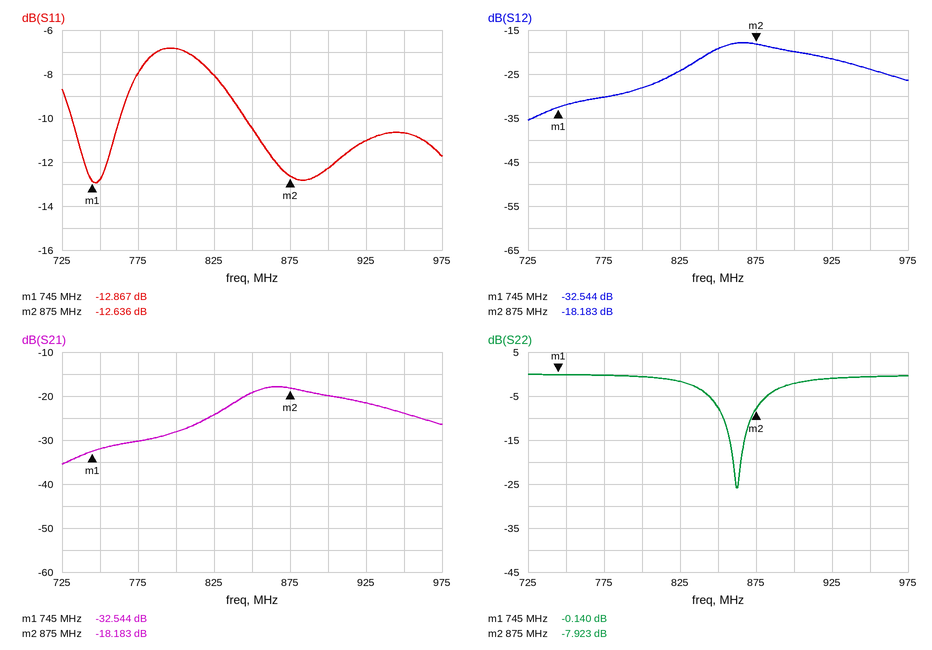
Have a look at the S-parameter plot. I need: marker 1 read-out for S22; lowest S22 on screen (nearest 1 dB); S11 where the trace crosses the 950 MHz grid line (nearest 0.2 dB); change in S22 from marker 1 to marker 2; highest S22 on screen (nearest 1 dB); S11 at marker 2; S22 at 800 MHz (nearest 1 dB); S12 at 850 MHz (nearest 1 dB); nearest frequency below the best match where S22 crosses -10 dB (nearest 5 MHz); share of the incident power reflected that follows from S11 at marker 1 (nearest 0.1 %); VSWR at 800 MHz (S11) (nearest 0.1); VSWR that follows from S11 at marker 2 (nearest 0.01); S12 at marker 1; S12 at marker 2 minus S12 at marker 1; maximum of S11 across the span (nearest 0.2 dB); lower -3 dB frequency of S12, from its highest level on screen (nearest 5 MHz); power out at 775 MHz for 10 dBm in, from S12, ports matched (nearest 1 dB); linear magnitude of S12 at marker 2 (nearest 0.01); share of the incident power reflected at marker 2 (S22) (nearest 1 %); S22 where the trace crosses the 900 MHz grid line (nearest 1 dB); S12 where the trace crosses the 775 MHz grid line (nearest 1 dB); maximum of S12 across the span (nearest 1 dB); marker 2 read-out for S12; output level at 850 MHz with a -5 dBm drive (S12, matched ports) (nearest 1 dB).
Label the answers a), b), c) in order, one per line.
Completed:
a) -0.140 dB
b) -26 dB
c) -10.6 dB
d) -7.783 dB
e) 0 dB
f) -12.636 dB
g) -1 dB
h) -19 dB
i) 855 MHz
j) 5.2 %
k) 2.7
l) 1.61
m) -32.544 dB
n) 14.361 dB
o) -6.8 dB
p) 840 MHz
q) -20 dBm
r) 0.12
s) 16 %
t) -2 dB
u) -30 dB
v) -18 dB
w) -18.183 dB
x) -24 dBm
